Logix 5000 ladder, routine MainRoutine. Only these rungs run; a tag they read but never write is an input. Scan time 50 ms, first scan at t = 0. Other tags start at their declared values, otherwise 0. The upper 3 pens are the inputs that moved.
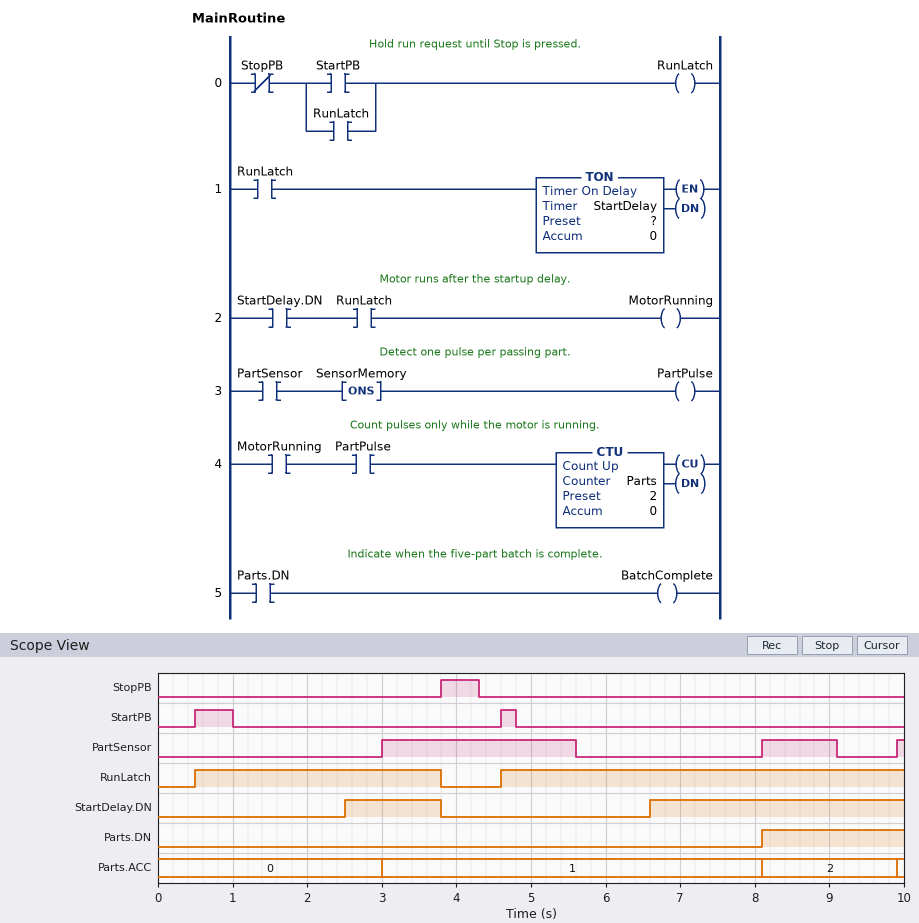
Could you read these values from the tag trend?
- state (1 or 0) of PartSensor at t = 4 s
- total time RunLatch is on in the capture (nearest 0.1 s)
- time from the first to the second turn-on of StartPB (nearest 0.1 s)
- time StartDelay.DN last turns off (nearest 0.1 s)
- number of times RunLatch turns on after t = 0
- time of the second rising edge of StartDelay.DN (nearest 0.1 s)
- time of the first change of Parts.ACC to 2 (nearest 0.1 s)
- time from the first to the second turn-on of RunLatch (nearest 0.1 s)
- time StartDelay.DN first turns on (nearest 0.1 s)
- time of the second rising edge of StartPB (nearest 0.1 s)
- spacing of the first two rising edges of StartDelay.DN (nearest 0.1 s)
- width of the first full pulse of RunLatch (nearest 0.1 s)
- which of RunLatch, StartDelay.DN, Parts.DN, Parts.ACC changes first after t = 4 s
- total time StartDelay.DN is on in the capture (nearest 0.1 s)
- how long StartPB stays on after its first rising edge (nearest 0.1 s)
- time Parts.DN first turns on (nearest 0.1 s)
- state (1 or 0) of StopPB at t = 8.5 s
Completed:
1
8.7 s
4.1 s
3.8 s
2
6.6 s
8.1 s
4.1 s
2.5 s
4.6 s
4.1 s
3.3 s
RunLatch
4.7 s
0.5 s
8.1 s
0
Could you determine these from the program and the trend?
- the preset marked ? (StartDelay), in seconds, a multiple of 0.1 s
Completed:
2.0 s
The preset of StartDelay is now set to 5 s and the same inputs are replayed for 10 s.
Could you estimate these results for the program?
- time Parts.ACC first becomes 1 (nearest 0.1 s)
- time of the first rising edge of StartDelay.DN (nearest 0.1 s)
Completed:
9.9 s
9.6 s
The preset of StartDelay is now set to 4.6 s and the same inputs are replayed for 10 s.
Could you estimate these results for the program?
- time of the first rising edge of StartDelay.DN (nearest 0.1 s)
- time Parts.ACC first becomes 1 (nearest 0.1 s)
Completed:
9.2 s
9.9 s
